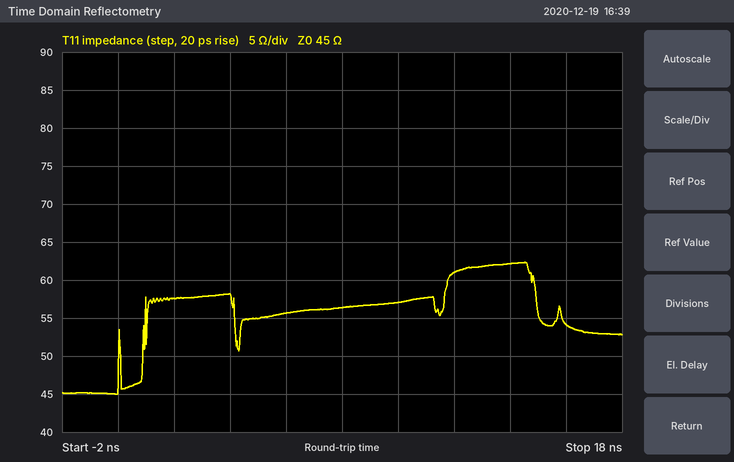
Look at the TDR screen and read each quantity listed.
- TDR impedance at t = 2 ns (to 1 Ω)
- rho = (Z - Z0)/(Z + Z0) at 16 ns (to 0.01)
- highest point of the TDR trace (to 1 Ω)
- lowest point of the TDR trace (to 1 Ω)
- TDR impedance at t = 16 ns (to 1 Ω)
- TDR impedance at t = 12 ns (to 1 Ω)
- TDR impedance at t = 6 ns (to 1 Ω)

58 Ω
+0.09
62 Ω
45 Ω
54 Ω
61 Ω
56 Ω
